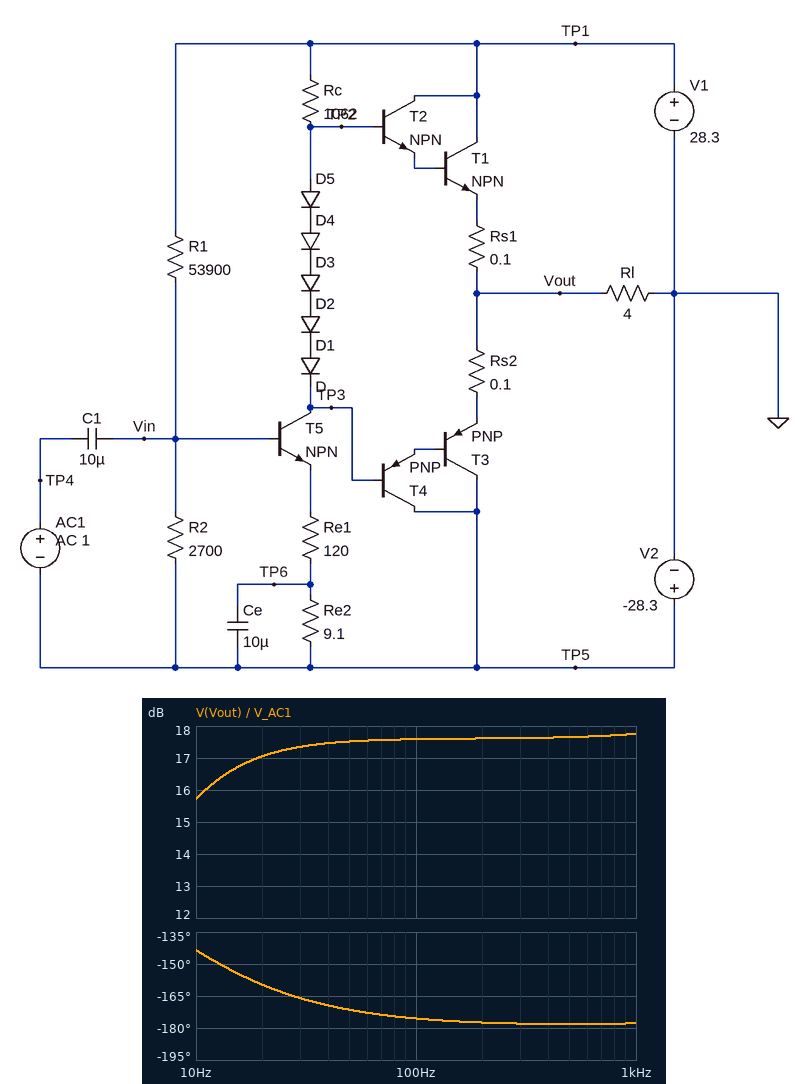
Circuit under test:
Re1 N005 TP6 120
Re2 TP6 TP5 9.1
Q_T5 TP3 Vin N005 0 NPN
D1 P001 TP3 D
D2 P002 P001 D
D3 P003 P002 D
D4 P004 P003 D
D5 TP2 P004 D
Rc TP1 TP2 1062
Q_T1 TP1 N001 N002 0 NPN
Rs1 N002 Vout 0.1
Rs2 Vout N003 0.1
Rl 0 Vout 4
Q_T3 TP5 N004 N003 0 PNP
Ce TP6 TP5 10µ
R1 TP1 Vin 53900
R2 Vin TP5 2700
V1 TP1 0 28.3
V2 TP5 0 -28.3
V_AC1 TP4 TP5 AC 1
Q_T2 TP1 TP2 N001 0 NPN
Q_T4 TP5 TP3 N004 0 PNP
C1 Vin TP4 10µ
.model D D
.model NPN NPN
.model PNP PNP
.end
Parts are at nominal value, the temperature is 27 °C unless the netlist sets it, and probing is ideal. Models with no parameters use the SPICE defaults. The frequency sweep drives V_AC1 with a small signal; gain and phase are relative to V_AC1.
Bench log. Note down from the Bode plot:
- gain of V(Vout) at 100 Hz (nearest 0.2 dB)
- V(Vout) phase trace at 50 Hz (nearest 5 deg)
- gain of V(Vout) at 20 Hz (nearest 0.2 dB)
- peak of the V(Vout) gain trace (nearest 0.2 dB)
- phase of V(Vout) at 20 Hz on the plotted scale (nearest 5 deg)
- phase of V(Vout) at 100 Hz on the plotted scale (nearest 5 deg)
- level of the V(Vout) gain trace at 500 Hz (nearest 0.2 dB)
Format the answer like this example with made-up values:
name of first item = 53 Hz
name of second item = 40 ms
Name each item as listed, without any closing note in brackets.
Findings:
gain of V(Vout) at 100 Hz = 17.6 dB
V(Vout) phase trace at 50 Hz = -170 deg
gain of V(Vout) at 20 Hz = 17.0 dB
peak of the V(Vout) gain trace = 17.8 dB
phase of V(Vout) at 20 Hz on the plotted scale = -160 deg
phase of V(Vout) at 100 Hz on the plotted scale = -175 deg
level of the V(Vout) gain trace at 500 Hz = 17.6 dB
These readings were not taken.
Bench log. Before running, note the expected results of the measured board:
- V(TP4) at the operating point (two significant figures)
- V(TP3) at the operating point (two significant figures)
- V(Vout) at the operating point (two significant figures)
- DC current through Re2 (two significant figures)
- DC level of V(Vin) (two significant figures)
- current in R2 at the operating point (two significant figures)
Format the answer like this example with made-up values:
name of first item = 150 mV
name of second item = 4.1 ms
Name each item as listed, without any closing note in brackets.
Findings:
V(TP4) at the operating point = -28 V
V(TP3) at the operating point = 12 V
V(Vout) at the operating point = 13 V
DC current through Re2 = 12 mA
DC level of V(Vin) = -26 V
current in R2 at the operating point = 890 µA
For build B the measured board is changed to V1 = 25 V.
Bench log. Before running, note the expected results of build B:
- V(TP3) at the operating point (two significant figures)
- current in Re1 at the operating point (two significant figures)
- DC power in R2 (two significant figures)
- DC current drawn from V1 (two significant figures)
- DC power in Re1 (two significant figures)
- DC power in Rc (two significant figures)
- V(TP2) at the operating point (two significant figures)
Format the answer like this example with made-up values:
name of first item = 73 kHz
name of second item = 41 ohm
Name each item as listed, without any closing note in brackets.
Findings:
V(TP3) at the operating point = 9.5 V
current in Re1 at the operating point = 11 mA
DC power in R2 = 1.9 mW
DC current drawn from V1 = 2.8 A
DC power in Re1 = 15 mW
DC power in Rc = 130 mW
V(TP2) at the operating point = 13 V
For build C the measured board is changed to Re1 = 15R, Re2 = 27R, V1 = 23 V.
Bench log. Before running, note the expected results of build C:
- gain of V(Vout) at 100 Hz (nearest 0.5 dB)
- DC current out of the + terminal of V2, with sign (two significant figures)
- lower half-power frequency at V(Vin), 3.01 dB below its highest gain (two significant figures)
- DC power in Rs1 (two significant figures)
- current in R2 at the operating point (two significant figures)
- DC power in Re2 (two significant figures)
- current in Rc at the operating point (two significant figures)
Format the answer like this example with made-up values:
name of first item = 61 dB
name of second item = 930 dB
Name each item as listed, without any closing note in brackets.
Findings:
gain of V(Vout) at 100 Hz = 27.5 dB
DC current out of the + terminal of V2, with sign = -1.2 A
lower half-power frequency at V(Vin), 3.01 dB below its highest gain = 9.9 Hz
DC power in Rs1 = 12 mW
current in R2 at the operating point = 680 µA
DC power in Re2 = 15 mW
current in Rc at the operating point = 23 mA
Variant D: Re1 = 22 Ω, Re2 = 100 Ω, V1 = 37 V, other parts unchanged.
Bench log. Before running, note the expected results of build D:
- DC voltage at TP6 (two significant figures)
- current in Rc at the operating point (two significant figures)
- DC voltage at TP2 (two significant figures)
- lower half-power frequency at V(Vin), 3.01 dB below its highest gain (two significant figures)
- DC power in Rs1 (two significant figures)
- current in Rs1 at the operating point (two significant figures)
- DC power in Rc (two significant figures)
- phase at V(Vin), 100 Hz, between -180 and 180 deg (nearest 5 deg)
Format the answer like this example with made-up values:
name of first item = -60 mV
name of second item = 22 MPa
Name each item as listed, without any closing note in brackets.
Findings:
DC voltage at TP6 = -27 V
current in Rc at the operating point = 16 mA
DC voltage at TP2 = 20 V
lower half-power frequency at V(Vin), 3.01 dB below its highest gain = 7.5 Hz
DC power in Rs1 = 2.0 W
current in Rs1 at the operating point = 4.5 A
DC power in Rc = 260 mW
phase at V(Vin), 100 Hz, between -180 and 180 deg = 5 deg
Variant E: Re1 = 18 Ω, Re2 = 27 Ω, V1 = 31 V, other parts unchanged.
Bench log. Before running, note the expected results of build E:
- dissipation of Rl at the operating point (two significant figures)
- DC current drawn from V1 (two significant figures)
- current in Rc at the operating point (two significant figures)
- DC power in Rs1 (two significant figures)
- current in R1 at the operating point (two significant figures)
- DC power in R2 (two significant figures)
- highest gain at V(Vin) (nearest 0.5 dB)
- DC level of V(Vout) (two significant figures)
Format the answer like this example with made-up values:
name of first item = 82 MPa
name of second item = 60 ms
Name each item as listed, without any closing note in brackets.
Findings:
dissipation of Rl at the operating point = 12 mW
DC current drawn from V1 = 790 mA
current in Rc at the operating point = 28 mA
DC power in Rs1 = 58 mW
current in R1 at the operating point = 1.1 mA
DC power in R2 = 1.7 mW
highest gain at V(Vin) = 0 dB
DC level of V(Vout) = -220 mV
